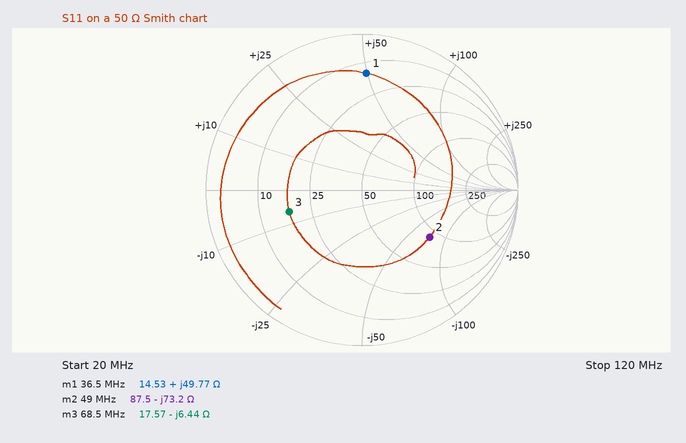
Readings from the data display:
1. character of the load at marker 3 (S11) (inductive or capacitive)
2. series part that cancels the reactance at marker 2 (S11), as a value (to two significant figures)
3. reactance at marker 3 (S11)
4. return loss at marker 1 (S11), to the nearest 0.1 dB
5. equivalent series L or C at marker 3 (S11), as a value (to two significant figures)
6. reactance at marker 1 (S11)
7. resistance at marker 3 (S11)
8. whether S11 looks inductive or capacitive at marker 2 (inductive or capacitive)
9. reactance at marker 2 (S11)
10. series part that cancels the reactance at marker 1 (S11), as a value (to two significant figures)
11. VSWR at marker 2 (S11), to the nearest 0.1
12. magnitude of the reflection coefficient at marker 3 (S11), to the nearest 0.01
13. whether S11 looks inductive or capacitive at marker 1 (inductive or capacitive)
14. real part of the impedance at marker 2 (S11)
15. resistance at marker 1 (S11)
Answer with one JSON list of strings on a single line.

["capacitive", "240 nH", "-6.44 Ω", "2.5 dB", "360 pF", "+49.77 Ω", "17.57 Ω", "capacitive", "-73.2 Ω", "88 pF", "3.2", "0.49", "inductive", "87.5 Ω", "14.53 Ω"]
